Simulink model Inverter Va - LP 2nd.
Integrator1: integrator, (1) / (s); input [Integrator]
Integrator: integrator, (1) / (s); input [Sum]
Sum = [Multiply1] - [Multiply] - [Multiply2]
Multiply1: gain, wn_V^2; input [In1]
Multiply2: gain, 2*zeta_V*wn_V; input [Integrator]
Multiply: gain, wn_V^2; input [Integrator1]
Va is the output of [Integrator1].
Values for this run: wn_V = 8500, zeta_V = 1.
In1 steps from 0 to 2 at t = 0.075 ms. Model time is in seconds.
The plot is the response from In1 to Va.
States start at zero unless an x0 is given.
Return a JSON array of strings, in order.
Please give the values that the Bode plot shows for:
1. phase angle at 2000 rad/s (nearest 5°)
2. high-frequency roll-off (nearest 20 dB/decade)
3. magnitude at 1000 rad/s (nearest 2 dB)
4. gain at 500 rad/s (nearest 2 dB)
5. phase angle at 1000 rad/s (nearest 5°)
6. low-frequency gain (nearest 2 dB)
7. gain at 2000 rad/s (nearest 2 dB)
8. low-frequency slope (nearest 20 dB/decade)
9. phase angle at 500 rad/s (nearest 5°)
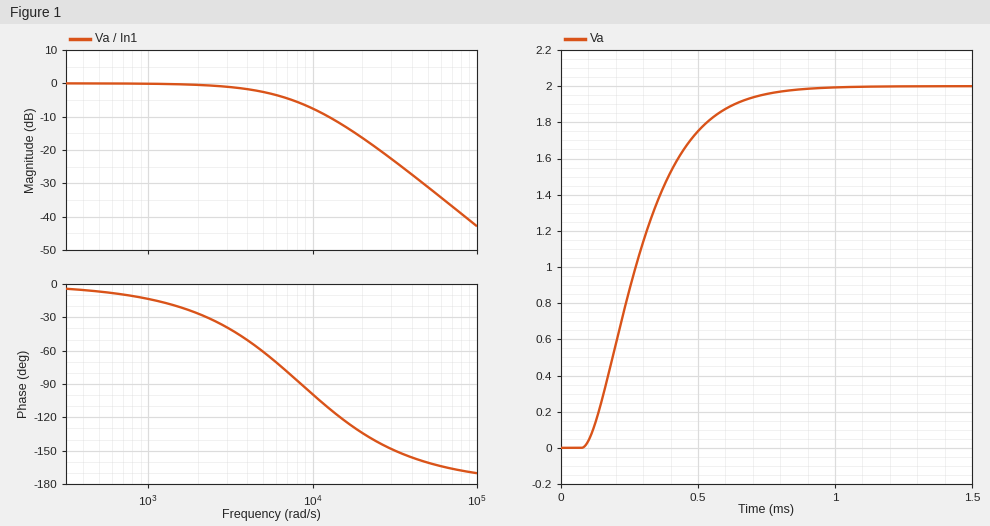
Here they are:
["-25°", "-40 dB/decade", "0 dB", "0 dB", "-15°", "0 dB", "0 dB", "0 dB/decade", "-5°"]
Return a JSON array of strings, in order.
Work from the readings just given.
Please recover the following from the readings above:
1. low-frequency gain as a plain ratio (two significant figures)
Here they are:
["1.0"]
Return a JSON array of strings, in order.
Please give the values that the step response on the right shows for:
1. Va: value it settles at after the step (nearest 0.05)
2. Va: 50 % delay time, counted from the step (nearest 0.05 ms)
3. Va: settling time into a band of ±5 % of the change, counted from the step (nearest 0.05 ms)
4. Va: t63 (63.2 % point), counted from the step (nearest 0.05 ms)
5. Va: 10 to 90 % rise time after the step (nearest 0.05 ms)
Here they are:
["2.00", "0.20 ms", "0.55 ms", "0.25 ms", "0.40 ms"]
